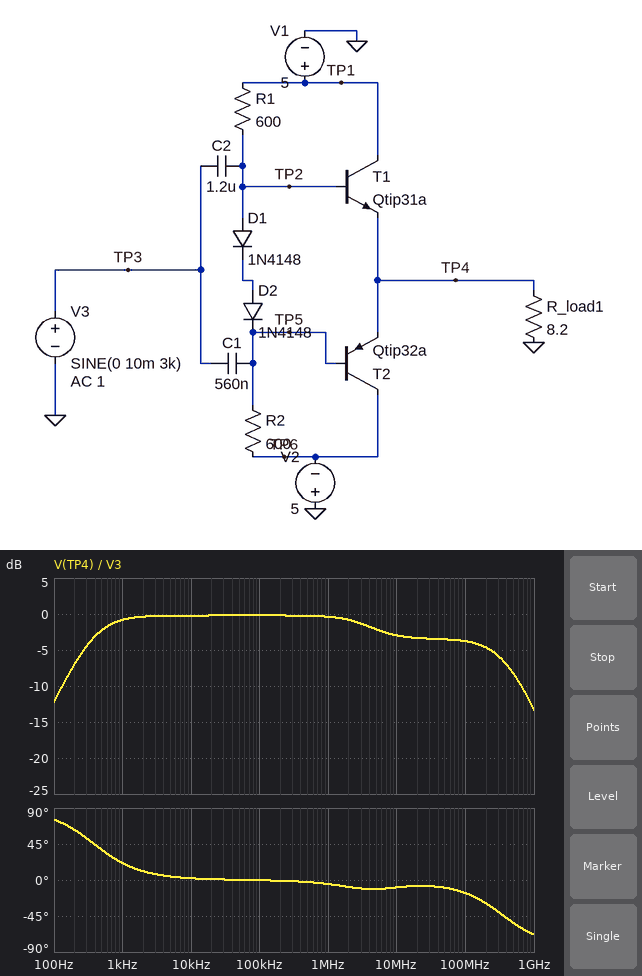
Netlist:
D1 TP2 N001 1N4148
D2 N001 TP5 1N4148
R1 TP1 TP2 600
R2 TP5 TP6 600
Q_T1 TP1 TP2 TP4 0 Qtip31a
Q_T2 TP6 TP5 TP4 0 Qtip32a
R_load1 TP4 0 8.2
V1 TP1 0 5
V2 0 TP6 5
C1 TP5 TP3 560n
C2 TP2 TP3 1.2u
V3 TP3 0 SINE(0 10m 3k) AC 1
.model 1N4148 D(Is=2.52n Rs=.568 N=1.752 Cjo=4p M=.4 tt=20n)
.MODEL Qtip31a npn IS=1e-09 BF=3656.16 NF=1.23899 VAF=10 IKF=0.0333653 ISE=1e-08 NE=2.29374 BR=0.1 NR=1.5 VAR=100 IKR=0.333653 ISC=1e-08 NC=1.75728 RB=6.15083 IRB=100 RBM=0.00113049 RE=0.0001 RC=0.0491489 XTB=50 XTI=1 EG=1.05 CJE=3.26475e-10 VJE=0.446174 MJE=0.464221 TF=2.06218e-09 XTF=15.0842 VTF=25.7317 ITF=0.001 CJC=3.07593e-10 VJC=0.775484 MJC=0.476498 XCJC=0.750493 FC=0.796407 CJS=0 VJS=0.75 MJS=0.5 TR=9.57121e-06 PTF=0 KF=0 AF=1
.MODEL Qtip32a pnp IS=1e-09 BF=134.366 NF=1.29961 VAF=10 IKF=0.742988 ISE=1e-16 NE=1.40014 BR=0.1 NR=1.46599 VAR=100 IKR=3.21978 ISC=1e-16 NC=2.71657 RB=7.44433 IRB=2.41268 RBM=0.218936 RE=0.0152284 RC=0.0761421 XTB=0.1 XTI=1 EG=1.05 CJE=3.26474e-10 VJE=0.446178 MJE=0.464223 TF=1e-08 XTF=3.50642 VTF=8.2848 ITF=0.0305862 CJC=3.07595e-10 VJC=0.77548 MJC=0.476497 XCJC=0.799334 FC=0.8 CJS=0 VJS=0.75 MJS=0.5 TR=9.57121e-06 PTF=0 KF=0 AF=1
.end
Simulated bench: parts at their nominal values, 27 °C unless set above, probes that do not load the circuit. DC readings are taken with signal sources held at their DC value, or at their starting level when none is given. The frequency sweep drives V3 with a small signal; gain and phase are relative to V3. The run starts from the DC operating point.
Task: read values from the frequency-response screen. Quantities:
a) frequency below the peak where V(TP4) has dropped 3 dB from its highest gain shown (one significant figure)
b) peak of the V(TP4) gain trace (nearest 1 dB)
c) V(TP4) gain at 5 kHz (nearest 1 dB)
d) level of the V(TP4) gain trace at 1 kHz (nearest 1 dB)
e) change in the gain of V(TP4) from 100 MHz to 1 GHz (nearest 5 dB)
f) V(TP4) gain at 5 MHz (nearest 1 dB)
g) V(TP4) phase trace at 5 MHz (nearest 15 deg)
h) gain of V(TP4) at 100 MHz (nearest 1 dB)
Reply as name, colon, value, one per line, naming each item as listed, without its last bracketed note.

frequency below the peak where V(TP4) has dropped 3 dB from its highest gain shown: 400 Hz
peak of the V(TP4) gain trace: 0 dB
V(TP4) gain at 5 kHz: 0 dB
level of the V(TP4) gain trace at 1 kHz: -1 dB
change in the gain of V(TP4) from 100 MHz to 1 GHz: -10 dB
V(TP4) gain at 5 MHz: -2 dB
V(TP4) phase trace at 5 MHz: -15 deg
gain of V(TP4) at 100 MHz: -4 dB
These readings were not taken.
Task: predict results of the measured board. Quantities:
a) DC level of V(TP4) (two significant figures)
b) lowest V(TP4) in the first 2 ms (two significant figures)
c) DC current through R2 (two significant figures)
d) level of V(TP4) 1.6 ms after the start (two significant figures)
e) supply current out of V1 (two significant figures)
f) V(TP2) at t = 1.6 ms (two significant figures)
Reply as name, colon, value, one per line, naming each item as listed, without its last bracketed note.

DC level of V(TP4): 120 mV
lowest V(TP4) in the first 2 ms: 110 mV
DC current through R2: 7.4 mA
level of V(TP4) 1.6 ms after the start: 110 mV
supply current out of V1: 270 mA
V(TP2) at t = 1.6 ms: 790 mV
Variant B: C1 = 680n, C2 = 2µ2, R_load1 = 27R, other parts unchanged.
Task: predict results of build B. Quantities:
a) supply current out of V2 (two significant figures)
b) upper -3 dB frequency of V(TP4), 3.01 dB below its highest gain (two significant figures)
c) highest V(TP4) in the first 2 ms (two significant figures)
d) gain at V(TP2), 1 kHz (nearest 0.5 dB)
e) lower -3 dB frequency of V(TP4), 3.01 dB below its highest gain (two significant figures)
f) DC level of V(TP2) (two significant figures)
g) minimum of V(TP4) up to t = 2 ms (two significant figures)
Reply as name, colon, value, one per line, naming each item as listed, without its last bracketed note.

supply current out of V2: 260 mA
upper -3 dB frequency of V(TP4), 3.01 dB below its highest gain: 190 MHz
highest V(TP4) in the first 2 ms: 150 mV
gain at V(TP2), 1 kHz: 0 dB
lower -3 dB frequency of V(TP4), 3.01 dB below its highest gain: 210 Hz
DC level of V(TP2): 810 mV
minimum of V(TP4) up to t = 2 ms: 130 mV
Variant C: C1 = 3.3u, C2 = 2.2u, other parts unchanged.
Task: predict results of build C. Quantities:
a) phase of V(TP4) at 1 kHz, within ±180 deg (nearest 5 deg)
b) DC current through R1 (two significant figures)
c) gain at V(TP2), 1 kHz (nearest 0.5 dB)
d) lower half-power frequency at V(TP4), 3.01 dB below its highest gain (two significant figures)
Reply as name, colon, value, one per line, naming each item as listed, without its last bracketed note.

phase of V(TP4) at 1 kHz, within ±180 deg: 5 deg
DC current through R1: 7.0 mA
gain at V(TP2), 1 kHz: 0 dB
lower half-power frequency at V(TP4), 3.01 dB below its highest gain: 130 Hz
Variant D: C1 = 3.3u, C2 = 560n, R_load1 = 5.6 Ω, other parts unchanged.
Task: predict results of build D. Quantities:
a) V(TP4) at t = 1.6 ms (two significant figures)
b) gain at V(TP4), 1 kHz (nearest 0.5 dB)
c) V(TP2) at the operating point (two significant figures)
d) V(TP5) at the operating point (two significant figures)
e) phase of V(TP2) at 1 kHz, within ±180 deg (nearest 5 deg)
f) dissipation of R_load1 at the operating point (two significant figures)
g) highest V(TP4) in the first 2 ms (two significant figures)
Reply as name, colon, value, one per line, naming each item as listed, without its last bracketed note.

V(TP4) at t = 1.6 ms: 100 mV
gain at V(TP4), 1 kHz: -0.5 dB
V(TP2) at the operating point: 790 mV
V(TP5) at the operating point: -550 mV
phase of V(TP2) at 1 kHz, within ±180 deg: 10 deg
dissipation of R_load1 at the operating point: 2.1 mW
highest V(TP4) in the first 2 ms: 120 mV
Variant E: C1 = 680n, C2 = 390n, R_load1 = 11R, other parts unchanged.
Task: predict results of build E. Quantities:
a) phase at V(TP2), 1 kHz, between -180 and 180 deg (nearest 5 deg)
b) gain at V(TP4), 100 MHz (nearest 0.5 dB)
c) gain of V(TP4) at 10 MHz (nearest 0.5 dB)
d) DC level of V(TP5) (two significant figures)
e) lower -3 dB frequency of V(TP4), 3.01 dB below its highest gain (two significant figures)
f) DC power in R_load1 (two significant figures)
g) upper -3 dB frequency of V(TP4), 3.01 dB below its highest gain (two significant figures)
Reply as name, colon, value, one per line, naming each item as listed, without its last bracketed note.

phase at V(TP2), 1 kHz, between -180 and 180 deg: 30 deg
gain at V(TP4), 100 MHz: -3.0 dB
gain of V(TP4) at 10 MHz: -2.5 dB
DC level of V(TP5): -530 mV
lower -3 dB frequency of V(TP4), 3.01 dB below its highest gain: 620 Hz
DC power in R_load1: 1.4 mW
upper -3 dB frequency of V(TP4), 3.01 dB below its highest gain: 98 MHz
